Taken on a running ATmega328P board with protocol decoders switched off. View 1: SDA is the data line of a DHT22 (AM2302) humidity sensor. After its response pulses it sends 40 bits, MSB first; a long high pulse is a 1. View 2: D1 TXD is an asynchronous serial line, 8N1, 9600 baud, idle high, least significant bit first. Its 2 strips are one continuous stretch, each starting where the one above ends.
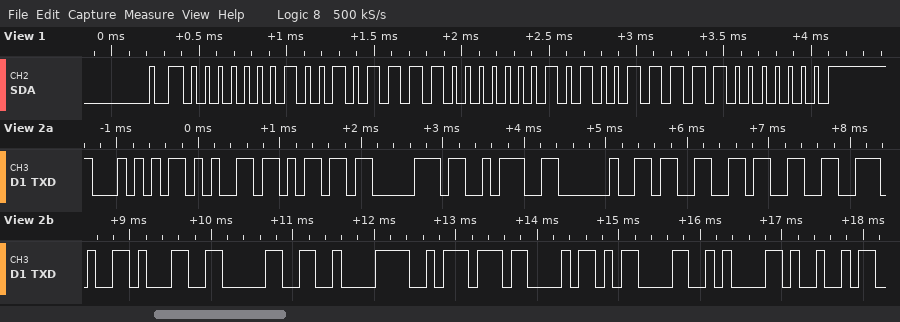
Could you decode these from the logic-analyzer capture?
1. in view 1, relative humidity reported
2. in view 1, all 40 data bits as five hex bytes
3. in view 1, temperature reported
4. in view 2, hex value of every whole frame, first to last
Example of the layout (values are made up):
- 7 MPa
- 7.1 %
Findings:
- 30.3 %
- 01 2F 01 4F 80
- 33.5 °C
- 54 65 6D 70 3A 20 33 33 2E 31 30 C2 BA 43 0D 0A 49
